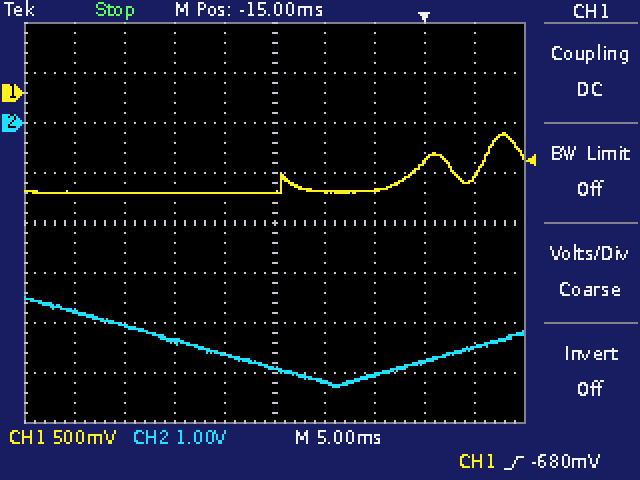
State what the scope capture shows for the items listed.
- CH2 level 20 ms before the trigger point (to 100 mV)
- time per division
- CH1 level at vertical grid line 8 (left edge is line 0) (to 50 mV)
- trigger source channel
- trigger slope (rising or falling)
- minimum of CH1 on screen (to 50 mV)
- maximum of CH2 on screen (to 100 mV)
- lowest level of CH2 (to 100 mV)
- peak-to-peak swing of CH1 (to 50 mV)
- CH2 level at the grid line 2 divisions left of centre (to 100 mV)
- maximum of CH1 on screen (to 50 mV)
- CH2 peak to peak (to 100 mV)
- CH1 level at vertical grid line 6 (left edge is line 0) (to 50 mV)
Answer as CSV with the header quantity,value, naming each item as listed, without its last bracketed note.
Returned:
quantity,value
CH2 level 20 ms before the trigger point,-4.6 V
time per division,5 ms
CH1 level at vertical grid line 8 (left edge is line 0),-700 mV
trigger source channel,CH1
trigger slope,rising
minimum of CH1 on screen,-1.00 V
maximum of CH2 on screen,-3.5 V
lowest level of CH2,-5.3 V
peak-to-peak swing of CH1,600 mV
CH2 level at the grid line 2 divisions left of centre,-4.4 V
maximum of CH1 on screen,-400 mV
CH2 peak to peak,1.8 V
CH1 level at vertical grid line 6 (left edge is line 0),-1.00 V
